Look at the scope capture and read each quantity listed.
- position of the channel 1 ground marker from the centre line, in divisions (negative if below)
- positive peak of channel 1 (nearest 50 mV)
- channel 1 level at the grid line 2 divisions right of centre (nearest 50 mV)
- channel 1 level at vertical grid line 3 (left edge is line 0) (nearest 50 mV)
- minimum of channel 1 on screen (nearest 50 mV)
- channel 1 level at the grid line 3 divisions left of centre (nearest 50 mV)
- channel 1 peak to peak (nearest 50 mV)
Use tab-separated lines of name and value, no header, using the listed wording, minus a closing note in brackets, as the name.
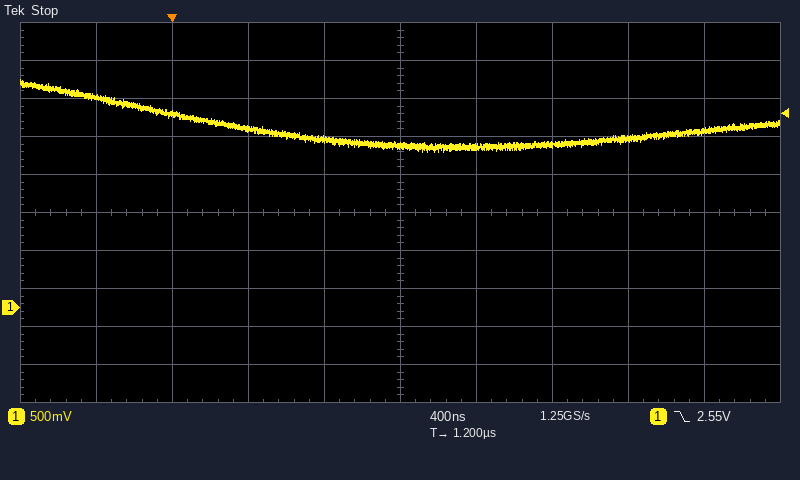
position of the channel 1 ground marker from the centre line, in divisions	-2.5 div
positive peak of channel 1	3.00 V
channel 1 level at the grid line 2 divisions right of centre	2.15 V
channel 1 level at vertical grid line 3 (left edge is line 0)	2.35 V
minimum of channel 1 on screen	2.05 V
channel 1 level at the grid line 3 divisions left of centre	2.55 V
channel 1 peak to peak	950 mV
